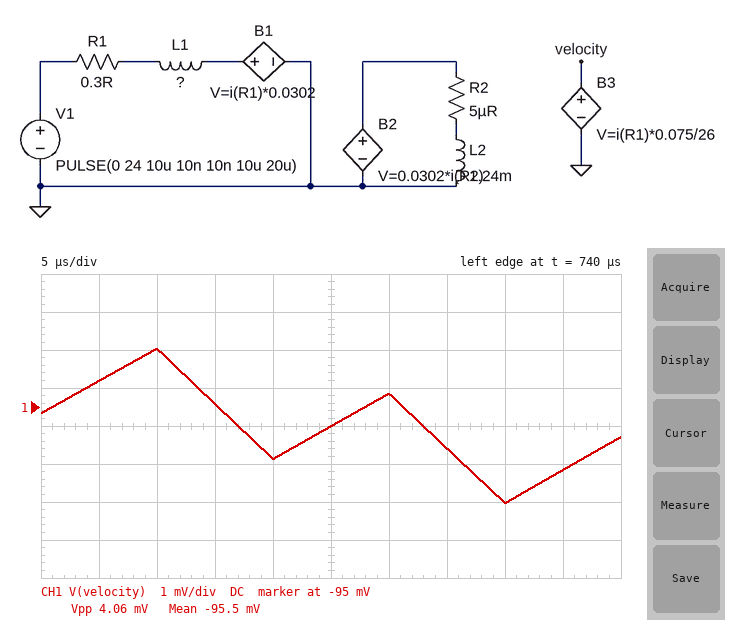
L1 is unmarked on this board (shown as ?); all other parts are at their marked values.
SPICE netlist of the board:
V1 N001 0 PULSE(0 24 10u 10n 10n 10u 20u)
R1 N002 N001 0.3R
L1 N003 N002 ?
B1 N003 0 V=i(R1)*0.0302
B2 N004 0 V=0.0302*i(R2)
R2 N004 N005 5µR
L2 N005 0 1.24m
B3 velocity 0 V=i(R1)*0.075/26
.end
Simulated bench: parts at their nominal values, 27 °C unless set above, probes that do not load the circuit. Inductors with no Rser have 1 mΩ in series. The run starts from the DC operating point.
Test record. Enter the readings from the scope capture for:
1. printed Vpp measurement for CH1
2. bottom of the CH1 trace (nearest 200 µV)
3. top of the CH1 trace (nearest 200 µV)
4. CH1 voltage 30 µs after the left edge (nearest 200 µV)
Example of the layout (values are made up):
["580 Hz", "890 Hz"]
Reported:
["4.06 mV", "-97.6 mV", "-93.4 mV", "-94.6 mV"]
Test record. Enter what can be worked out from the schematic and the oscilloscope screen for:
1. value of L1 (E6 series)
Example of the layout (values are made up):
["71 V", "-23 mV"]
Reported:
["150 µH"]
